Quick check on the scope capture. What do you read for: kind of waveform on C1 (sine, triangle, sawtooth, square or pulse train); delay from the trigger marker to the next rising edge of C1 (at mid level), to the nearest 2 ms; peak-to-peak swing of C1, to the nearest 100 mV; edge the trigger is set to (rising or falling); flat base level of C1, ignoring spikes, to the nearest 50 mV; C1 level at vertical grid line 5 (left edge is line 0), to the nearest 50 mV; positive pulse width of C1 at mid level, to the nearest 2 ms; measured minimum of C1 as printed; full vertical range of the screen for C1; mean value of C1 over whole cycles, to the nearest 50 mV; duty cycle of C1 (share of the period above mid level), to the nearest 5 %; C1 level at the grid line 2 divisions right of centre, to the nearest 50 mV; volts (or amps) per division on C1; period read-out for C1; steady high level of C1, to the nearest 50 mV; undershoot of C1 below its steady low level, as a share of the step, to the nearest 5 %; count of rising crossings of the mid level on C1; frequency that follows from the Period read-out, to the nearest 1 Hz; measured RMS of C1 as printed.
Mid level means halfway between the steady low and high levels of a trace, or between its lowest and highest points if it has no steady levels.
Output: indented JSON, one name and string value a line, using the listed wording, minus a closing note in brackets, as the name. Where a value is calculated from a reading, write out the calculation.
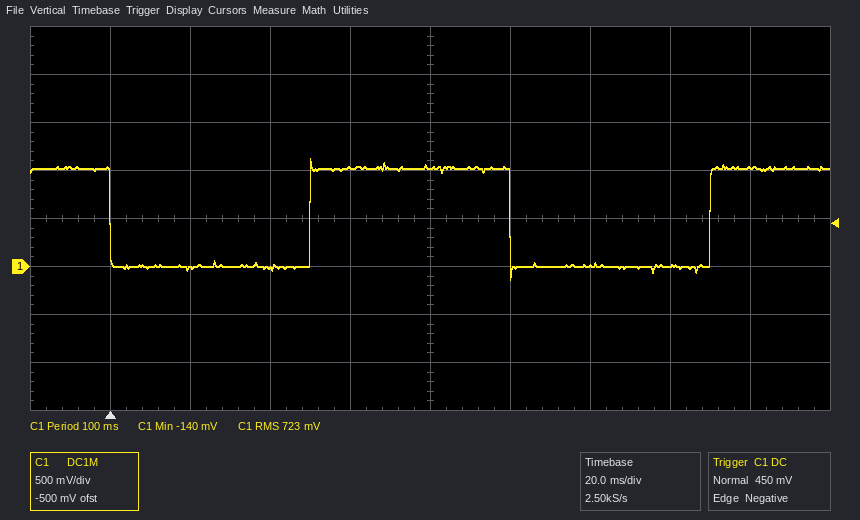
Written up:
{
  "kind of waveform on C1": "square",
  "delay from the trigger marker to the next rising edge of C1 (at mid level), to the nearest 2 ms": "50 ms",
  "peak-to-peak swing of C1, to the nearest 100 mV": "1.30 V",
  "edge the trigger is set to": "falling",
  "flat base level of C1, ignoring spikes, to the nearest 50 mV": "0 mV",
  "C1 level at vertical grid line 5 (left edge is line 0), to the nearest 50 mV": "1.05 V",
  "positive pulse width of C1 at mid level, to the nearest 2 ms": "50 ms",
  "measured minimum of C1 as printed": "-140 mV",
  "full vertical range of the screen for C1": "4 V",
  "mean value of C1 over whole cycles, to the nearest 50 mV": "0 mV + 0.5 × (1.00 V − (0 mV)) ≈ 500 mV",
  "duty cycle of C1 (share of the period above mid level), to the nearest 5 %": "50 %",
  "C1 level at the grid line 2 divisions right of centre, to the nearest 50 mV": "0 mV",
  "volts (or amps) per division on C1": "500 mV",
  "period read-out for C1": "100 ms",
  "steady high level of C1, to the nearest 50 mV": "1.00 V",
  "undershoot of C1 below its steady low level, as a share of the step, to the nearest 5 %": "15 %",
  "count of rising crossings of the mid level on C1": "2",
  "frequency that follows from the Period read-out, to the nearest 1 Hz": "1 / 100 ms ≈ 10 Hz",
  "measured RMS of C1 as printed": "723 mV"
}
